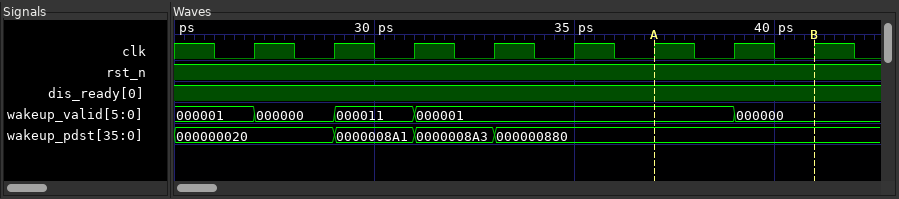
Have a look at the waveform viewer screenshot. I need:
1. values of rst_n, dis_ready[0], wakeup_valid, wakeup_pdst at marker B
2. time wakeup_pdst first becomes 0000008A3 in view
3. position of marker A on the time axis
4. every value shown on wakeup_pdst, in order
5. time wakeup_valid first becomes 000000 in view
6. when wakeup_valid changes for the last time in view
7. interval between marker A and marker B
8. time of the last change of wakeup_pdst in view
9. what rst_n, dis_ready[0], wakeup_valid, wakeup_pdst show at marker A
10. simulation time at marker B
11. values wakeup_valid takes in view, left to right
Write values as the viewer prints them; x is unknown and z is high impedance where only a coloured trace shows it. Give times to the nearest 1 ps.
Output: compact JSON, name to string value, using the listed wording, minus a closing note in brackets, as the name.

{"values of rst_n, dis_ready[0], wakeup_valid, wakeup_pdst at marker B": "rst_n=1, dis_ready[0]=1, wakeup_valid=000000, wakeup_pdst=000000880", "time wakeup_pdst first becomes 0000008A3 in view": "31 ps", "position of marker A on the time axis": "37 ps", "every value shown on wakeup_pdst, in order": "000000020, 0000008A1, 0000008A3, 000000880", "time wakeup_valid first becomes 000000 in view": "27 ps", "when wakeup_valid changes for the last time in view": "39 ps", "interval between marker A and marker B": "4 ps", "time of the last change of wakeup_pdst in view": "33 ps", "what rst_n, dis_ready[0], wakeup_valid, wakeup_pdst show at marker A": "rst_n=1, dis_ready[0]=1, wakeup_valid=000001, wakeup_pdst=000000880", "simulation time at marker B": "41 ps", "values wakeup_valid takes in view, left to right": "000001, 000000, 000011, 000001, 000000"}
